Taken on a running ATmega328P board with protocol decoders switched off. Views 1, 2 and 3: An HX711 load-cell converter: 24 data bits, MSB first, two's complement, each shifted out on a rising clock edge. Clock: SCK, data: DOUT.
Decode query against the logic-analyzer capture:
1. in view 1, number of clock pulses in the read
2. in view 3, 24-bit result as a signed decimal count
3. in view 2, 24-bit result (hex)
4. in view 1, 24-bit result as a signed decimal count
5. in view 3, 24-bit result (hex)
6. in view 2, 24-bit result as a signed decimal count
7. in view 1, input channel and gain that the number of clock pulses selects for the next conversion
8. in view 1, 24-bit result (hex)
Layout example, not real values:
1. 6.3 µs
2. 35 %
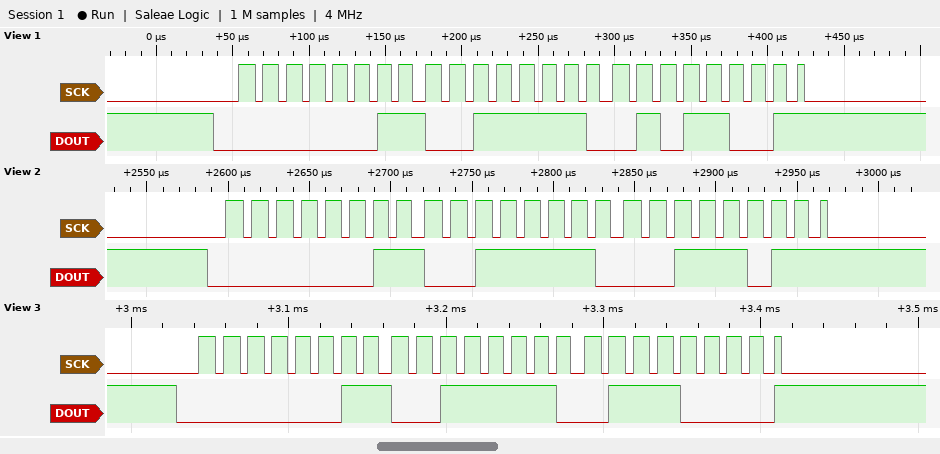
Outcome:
1. 25
2. 212592
3. 0x033E3B
4. 212569
5. 0x033E70
6. 212539
7. channel A, gain 128
8. 0x033E59
